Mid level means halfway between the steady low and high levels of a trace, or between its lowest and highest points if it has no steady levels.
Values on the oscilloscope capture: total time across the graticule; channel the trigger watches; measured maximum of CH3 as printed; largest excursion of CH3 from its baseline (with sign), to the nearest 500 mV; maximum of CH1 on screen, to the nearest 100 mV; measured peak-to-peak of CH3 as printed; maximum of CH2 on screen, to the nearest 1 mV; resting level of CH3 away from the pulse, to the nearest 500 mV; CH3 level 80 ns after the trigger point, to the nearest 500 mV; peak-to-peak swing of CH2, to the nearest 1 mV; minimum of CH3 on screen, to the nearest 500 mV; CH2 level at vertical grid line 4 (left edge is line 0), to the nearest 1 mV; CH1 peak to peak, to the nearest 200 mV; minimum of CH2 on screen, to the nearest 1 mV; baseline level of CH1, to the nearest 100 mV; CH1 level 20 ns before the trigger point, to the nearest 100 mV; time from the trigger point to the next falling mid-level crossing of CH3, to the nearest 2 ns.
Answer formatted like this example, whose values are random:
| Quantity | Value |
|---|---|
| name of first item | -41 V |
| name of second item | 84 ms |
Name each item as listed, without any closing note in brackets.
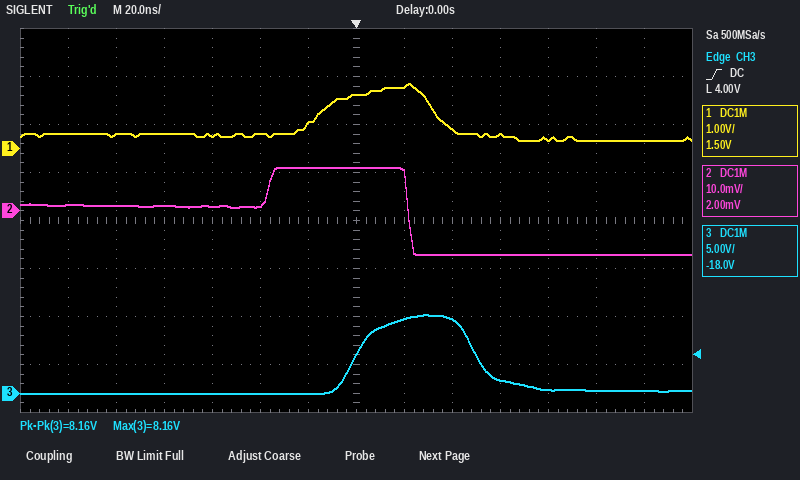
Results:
| Quantity | Value |
|---|---|
| total time across the graticule | 280 ns |
| channel the trigger watches | CH3 |
| measured maximum of CH3 as printed | 8.16 V |
| largest excursion of CH3 from its baseline (with sign), to the nearest 500 mV | +8.0 V |
| maximum of CH1 on screen, to the nearest 100 mV | 1.4 V |
| measured peak-to-peak of CH3 as printed | 8.16 V |
| maximum of CH2 on screen, to the nearest 1 mV | 9 mV |
| resting level of CH3 away from the pulse, to the nearest 500 mV | 0.0 V |
| CH3 level 80 ns after the trigger point, to the nearest 500 mV | 500 mV |
| peak-to-peak swing of CH2, to the nearest 1 mV | 18 mV |
| minimum of CH3 on screen, to the nearest 500 mV | 0.0 V |
| CH2 level at vertical grid line 4 (left edge is line 0), to the nearest 1 mV | 1 mV |
| CH1 peak to peak, to the nearest 200 mV | 1.2 V |
| minimum of CH2 on screen, to the nearest 1 mV | -9 mV |
| baseline level of CH1, to the nearest 100 mV | 300 mV |
| CH1 level 20 ns before the trigger point, to the nearest 100 mV | 500 mV |
| time from the trigger point to the next falling mid-level crossing of CH3, to the nearest 2 ns | 50 ns |
